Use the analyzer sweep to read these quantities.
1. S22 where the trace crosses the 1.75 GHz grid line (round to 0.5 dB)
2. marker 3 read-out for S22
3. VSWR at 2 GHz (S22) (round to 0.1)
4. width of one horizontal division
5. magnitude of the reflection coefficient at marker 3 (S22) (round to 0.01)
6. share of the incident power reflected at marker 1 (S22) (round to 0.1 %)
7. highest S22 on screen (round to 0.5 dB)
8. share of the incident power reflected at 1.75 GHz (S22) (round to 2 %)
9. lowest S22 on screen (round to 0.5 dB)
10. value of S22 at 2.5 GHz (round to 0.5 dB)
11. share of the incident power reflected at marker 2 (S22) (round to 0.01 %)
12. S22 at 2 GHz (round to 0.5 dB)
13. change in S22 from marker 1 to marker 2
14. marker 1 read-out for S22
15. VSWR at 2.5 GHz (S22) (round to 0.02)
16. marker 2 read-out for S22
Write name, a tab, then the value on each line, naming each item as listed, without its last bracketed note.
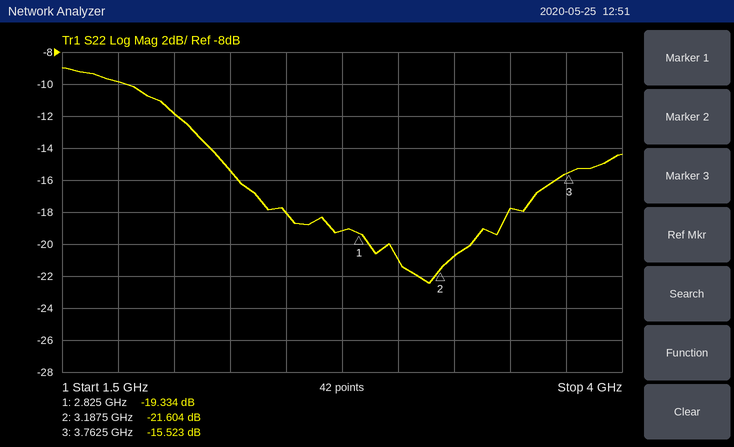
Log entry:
S22 where the trace crosses the 1.75 GHz grid line	-10.0 dB
marker 3 read-out for S22	-15.523 dB
VSWR at 2 GHz (S22)	1.7
width of one horizontal division	250 MHz
magnitude of the reflection coefficient at marker 3 (S22)	0.17
share of the incident power reflected at marker 1 (S22)	1.2 %
highest S22 on screen	-9.0 dB
share of the incident power reflected at 1.75 GHz (S22)	10 %
lowest S22 on screen	-22.5 dB
value of S22 at 2.5 GHz	-18.0 dB
share of the incident power reflected at marker 2 (S22)	0.69 %
S22 at 2 GHz	-12.0 dB
change in S22 from marker 1 to marker 2	-2.270 dB
marker 1 read-out for S22	-19.334 dB
VSWR at 2.5 GHz (S22)	1.28
marker 2 read-out for S22	-21.604 dB
